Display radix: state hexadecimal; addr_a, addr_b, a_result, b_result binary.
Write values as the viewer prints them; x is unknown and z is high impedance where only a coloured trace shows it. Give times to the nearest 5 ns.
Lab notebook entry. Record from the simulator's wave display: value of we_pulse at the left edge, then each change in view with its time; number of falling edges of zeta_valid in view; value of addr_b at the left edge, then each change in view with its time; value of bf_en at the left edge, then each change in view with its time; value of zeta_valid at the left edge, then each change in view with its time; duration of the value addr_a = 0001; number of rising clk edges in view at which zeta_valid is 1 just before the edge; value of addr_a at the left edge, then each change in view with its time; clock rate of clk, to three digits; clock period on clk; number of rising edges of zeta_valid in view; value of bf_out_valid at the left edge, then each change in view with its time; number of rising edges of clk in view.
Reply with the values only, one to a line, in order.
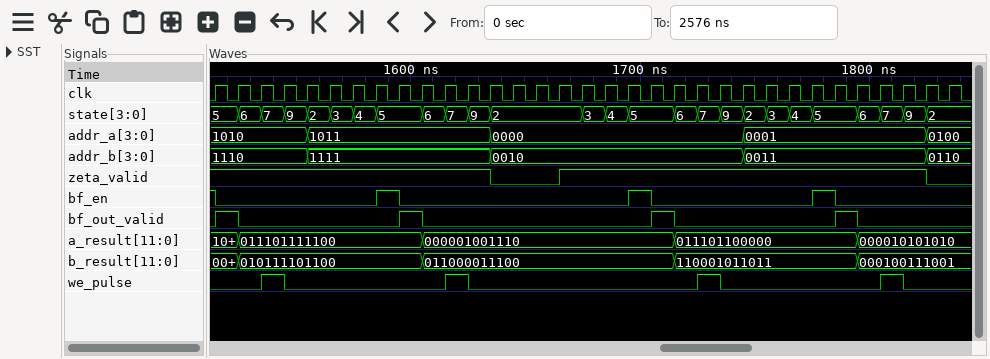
0, 1 at 1535 ns, 0 at 1545 ns, 1 at 1615 ns, 0 at 1625 ns, 1 at 1725 ns, 0 at 1735 ns, 1 at 1805 ns, 0 at 1815 ns
2
1110, 1111 at 1555 ns, 0010 at 1635 ns, 0011 at 1745 ns, 0110 at 1825 ns
1, 0 at 1515 ns, 1 at 1585 ns, 0 at 1595 ns, 1 at 1695 ns, 0 at 1705 ns, 1 at 1775 ns, 0 at 1785 ns
1, 0 at 1635 ns, 1 at 1665 ns, 0 at 1825 ns
80 ns
29
1010, 1011 at 1555 ns, 0000 at 1635 ns, 0001 at 1745 ns, 0100 at 1825 ns
100 MHz
10 ns
1
0, 1 at 1515 ns, 0 at 1525 ns, 1 at 1595 ns, 0 at 1605 ns, 1 at 1705 ns, 0 at 1715 ns, 1 at 1785 ns, 0 at 1795 ns
33
